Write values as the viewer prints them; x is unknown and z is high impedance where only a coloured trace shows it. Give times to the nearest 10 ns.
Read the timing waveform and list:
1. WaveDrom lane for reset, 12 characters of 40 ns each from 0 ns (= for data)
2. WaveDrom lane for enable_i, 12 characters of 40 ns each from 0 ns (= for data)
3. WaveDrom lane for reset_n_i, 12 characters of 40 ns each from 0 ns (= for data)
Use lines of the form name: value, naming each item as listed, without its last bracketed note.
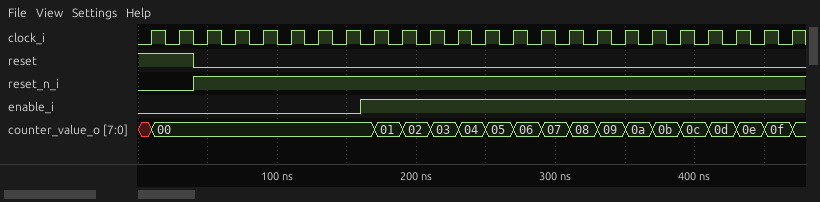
WaveDrom lane for reset, 12 characters of 40 ns each from 0 ns: {name: 'reset', wave: '10..........'}
WaveDrom lane for enable_i, 12 characters of 40 ns each from 0 ns: {name: 'enable_i', wave: '0...1.......'}
WaveDrom lane for reset_n_i, 12 characters of 40 ns each from 0 ns: {name: 'reset_n_i', wave: '01..........'}
